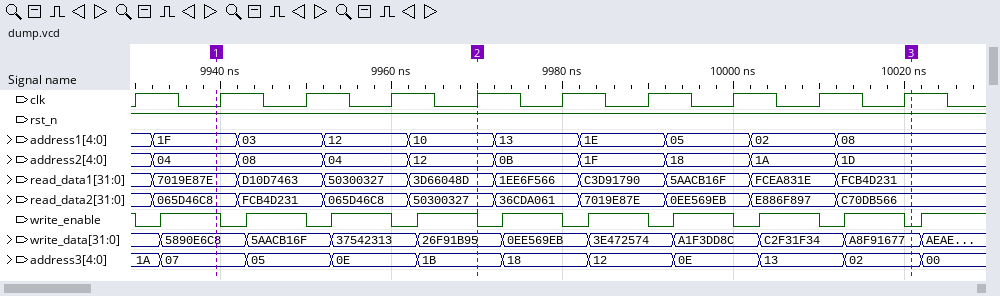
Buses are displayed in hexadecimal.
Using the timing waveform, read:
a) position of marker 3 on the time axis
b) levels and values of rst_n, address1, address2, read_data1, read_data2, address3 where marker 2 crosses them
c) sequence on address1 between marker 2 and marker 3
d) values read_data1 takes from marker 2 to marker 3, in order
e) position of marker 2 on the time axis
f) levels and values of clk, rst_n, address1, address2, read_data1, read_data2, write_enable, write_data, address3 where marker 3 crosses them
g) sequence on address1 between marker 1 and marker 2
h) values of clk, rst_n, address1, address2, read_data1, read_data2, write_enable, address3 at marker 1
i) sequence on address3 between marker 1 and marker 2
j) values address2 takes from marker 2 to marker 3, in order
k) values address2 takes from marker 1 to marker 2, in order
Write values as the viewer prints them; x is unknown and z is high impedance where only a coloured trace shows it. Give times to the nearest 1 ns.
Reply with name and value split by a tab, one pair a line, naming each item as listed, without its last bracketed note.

position of marker 3 on the time axis	10021 ns
levels and values of rst_n, address1, address2, read_data1, read_data2, address3 where marker 2 crosses them	rst_n=1, address1=10, address2=12, read_data1=3D66048D, read_data2=50300327, address3=1B
sequence on address1 between marker 2 and marker 3	10, 13, 1E, 05, 02, 08
values read_data1 takes from marker 2 to marker 3, in order	3D66048D, 1EE6F566, C3D91790, 5AACB16F, FCEA831E, FCB4D231
position of marker 2 on the time axis	9970 ns
levels and values of clk, rst_n, address1, address2, read_data1, read_data2, write_enable, write_data, address3 where marker 3 crosses them	clk=1, rst_n=1, address1=08, address2=1D, read_data1=FCB4D231, read_data2=C70DB566, write_enable=0, write_data=A8F91677, address3=02
sequence on address1 between marker 1 and marker 2	1F, 03, 12, 10
values of clk, rst_n, address1, address2, read_data1, read_data2, write_enable, address3 at marker 1	clk=0, rst_n=1, address1=1F, address2=04, read_data1=7019E87E, read_data2=065D46C8, write_enable=1, address3=07
sequence on address3 between marker 1 and marker 2	07, 05, 0E, 1B
values address2 takes from marker 2 to marker 3, in order	12, 0B, 1F, 18, 1A, 1D
values address2 takes from marker 1 to marker 2, in order	04, 08, 04, 12
